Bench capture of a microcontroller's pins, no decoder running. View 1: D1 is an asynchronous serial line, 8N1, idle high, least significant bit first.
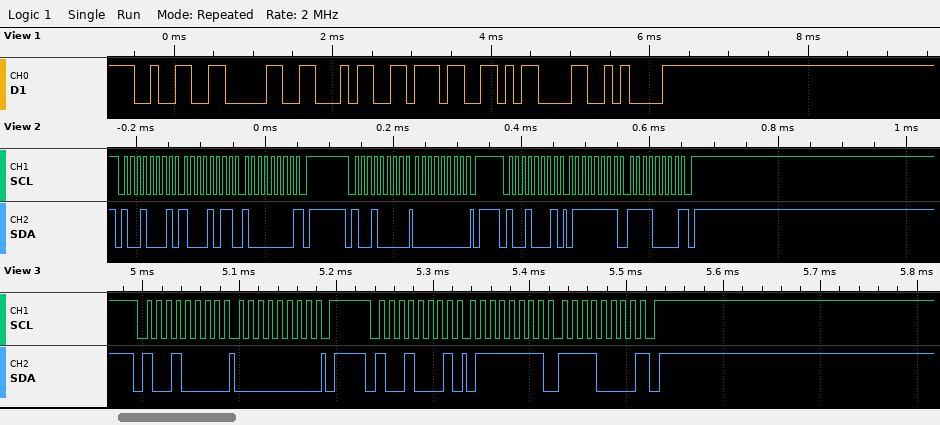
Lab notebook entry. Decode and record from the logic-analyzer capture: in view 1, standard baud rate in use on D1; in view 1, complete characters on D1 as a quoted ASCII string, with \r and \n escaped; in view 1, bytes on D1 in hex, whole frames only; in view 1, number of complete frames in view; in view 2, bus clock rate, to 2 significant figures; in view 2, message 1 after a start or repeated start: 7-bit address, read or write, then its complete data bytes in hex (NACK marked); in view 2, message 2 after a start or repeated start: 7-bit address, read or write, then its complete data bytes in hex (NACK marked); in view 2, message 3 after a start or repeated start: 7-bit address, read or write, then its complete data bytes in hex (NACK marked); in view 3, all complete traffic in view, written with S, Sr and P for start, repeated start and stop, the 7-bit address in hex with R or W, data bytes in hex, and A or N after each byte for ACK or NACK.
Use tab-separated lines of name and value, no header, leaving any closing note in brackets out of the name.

in view 1, standard baud rate in use on D1	9600 baud
in view 1, complete characters on D1 as a quoted ASCII string, with \r and \n escaped	"2047\r\n"
in view 1, bytes on D1 in hex, whole frames only	32 30 34 37 0D 0A
in view 1, number of complete frames in view	6
in view 2, bus clock rate, to 2 significant figures	100 kHz
in view 2, message 1 after a start or repeated start: 7-bit address, read or write, then its complete data bytes in hex	0x48 read: 8B 80 NACK
in view 2, message 2 after a start or repeated start: 7-bit address, read or write, then its complete data bytes in hex	0x48 write: 00
in view 2, message 3 after a start or repeated start: 7-bit address, read or write, then its complete data bytes in hex	0x48 read: 7F F0 NACK
in view 3, all complete traffic in view, written with S, Sr and P for start, repeated start and stop, the 7-bit address in hex with R or W, data bytes in hex, and A or N after each byte for ACK or NACK	S 48W A 00 A P S 48R A 7F A F0 N P
